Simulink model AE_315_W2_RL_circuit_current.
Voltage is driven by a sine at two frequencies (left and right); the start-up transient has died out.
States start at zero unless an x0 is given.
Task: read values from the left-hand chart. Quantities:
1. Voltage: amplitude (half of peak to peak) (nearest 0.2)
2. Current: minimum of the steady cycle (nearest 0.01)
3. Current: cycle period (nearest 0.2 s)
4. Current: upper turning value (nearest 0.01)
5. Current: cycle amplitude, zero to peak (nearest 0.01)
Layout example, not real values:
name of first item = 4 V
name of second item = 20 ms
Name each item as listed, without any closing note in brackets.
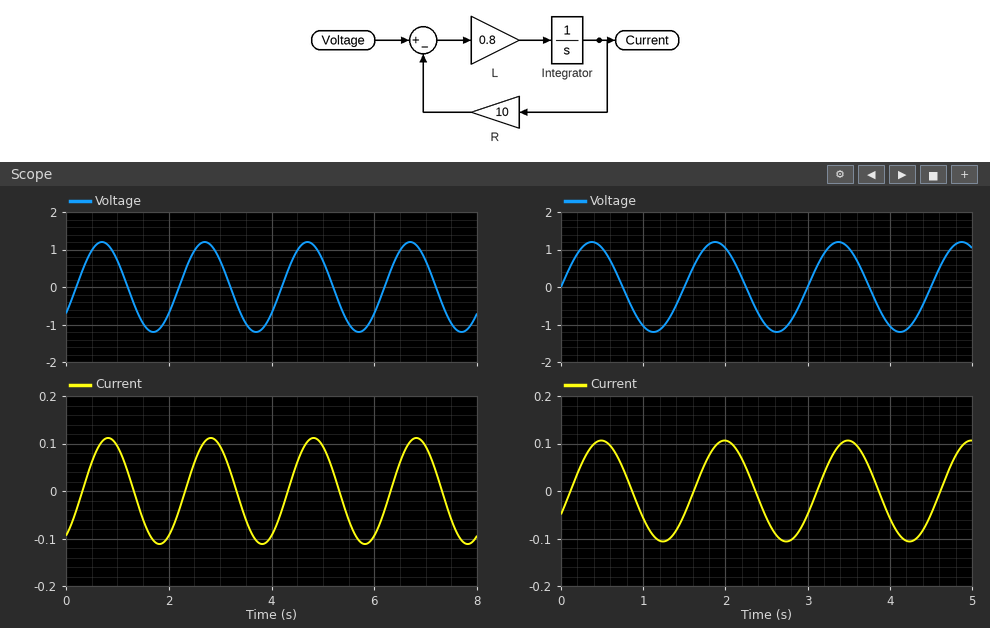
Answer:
Voltage: amplitude (half of peak to peak) = 1.2
Current: minimum of the steady cycle = -0.11
Current: cycle period = 2.0 s
Current: upper turning value = 0.11
Current: cycle amplitude, zero to peak = 0.11
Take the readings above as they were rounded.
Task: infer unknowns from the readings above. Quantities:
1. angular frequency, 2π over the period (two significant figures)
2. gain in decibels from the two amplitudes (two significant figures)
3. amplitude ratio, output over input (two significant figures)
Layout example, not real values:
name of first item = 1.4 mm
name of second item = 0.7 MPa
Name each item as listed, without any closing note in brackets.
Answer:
angular frequency, 2π over the period = 3.1 rad/s
gain in decibels from the two amplitudes = -21 dB
amplitude ratio, output over input = 0.092
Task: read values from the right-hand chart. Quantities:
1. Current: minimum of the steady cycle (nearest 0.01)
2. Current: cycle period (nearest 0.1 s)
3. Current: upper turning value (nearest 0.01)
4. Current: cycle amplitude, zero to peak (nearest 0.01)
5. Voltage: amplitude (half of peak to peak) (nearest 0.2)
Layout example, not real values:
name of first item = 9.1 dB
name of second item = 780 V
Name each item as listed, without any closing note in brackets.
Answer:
Current: minimum of the steady cycle = -0.11
Current: cycle period = 1.5 s
Current: upper turning value = 0.11
Current: cycle amplitude, zero to peak = 0.11
Voltage: amplitude (half of peak to peak) = 1.2
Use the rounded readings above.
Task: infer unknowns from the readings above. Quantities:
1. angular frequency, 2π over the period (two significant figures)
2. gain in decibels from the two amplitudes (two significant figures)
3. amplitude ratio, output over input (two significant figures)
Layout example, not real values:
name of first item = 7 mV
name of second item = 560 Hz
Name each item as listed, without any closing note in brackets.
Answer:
angular frequency, 2π over the period = 4.2 rad/s
gain in decibels from the two amplitudes = -21 dB
amplitude ratio, output over input = 0.092
